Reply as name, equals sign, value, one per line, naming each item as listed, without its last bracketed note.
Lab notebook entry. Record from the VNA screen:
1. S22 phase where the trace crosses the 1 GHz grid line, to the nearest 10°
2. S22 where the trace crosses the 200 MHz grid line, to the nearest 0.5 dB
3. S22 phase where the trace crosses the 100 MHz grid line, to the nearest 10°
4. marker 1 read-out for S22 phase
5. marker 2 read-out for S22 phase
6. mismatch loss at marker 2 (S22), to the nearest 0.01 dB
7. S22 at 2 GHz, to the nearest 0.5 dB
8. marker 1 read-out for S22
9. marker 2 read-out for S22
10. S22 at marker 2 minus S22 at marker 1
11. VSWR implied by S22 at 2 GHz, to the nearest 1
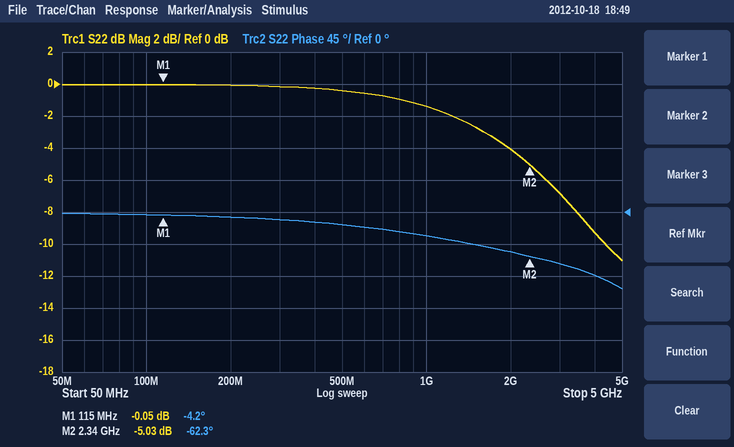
S22 phase where the trace crosses the 1 GHz grid line, to the nearest 10° = -30°
S22 where the trace crosses the 200 MHz grid line, to the nearest 0.5 dB = 0.0 dB
S22 phase where the trace crosses the 100 MHz grid line, to the nearest 10° = 0°
marker 1 read-out for S22 phase = -4.2°
marker 2 read-out for S22 phase = -62.3°
mismatch loss at marker 2 (S22), to the nearest 0.01 dB = 1.64 dB
S22 at 2 GHz, to the nearest 0.5 dB = -4.0 dB
marker 1 read-out for S22 = -0.05 dB
marker 2 read-out for S22 = -5.03 dB
S22 at marker 2 minus S22 at marker 1 = -4.98 dB
VSWR implied by S22 at 2 GHz, to the nearest 1 = 4
